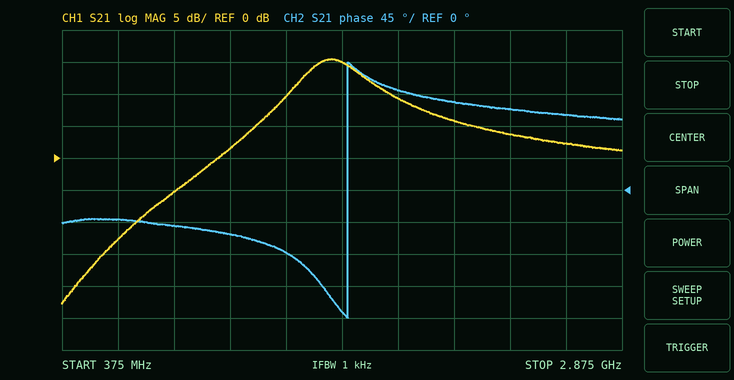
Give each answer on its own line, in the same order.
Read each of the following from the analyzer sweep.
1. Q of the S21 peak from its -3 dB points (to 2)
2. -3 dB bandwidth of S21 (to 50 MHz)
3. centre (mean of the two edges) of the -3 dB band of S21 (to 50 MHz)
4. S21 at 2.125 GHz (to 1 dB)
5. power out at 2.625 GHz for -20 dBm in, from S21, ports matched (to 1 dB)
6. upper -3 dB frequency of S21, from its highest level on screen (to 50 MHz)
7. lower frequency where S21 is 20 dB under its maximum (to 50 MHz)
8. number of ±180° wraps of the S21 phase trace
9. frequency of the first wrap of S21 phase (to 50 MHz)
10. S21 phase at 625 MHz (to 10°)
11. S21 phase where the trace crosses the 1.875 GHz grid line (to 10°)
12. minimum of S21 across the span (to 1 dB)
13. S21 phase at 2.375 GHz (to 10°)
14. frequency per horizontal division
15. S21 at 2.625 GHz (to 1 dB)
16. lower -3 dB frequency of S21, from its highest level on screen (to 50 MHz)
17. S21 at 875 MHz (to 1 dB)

6
300 MHz
1.60 GHz
6 dB
-18 dBm
1.75 GHz
900 MHz
1
1.65 GHz
-40°
140°
-23 dB
110°
250 MHz
2 dB
1.45 GHz
-5 dB
